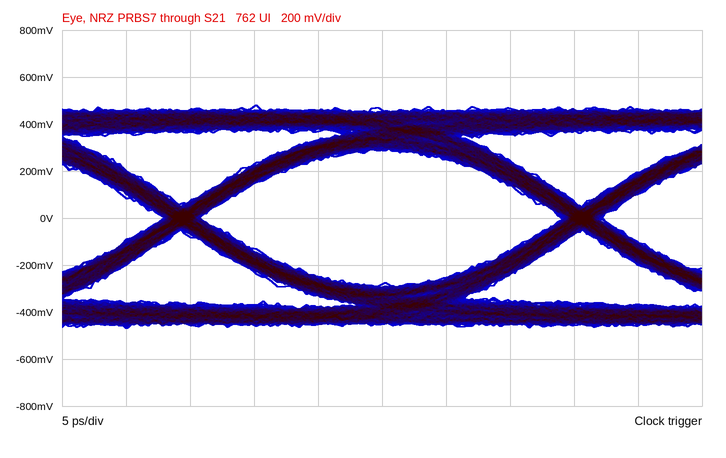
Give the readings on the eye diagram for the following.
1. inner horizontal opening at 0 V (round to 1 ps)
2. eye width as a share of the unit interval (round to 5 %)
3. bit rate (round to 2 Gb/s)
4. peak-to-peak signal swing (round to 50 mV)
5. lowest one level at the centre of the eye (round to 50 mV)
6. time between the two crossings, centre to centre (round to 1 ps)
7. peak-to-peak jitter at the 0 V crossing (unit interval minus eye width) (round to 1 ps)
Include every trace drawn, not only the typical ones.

28 ps
90 %
32 Gb/s
950 mV
300 mV
31 ps
3 ps
